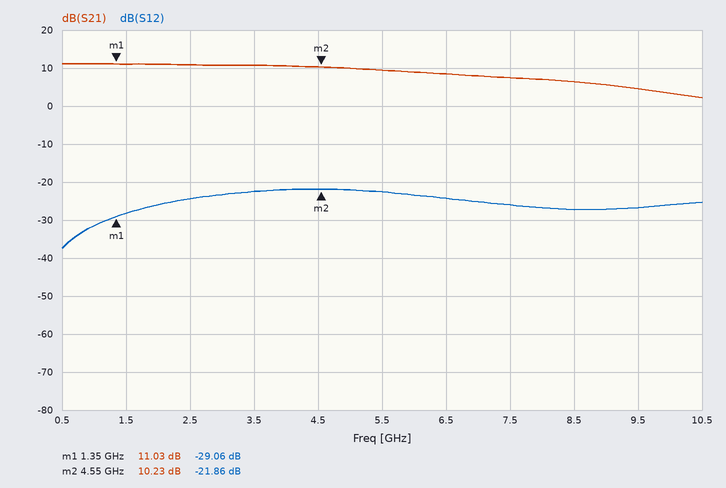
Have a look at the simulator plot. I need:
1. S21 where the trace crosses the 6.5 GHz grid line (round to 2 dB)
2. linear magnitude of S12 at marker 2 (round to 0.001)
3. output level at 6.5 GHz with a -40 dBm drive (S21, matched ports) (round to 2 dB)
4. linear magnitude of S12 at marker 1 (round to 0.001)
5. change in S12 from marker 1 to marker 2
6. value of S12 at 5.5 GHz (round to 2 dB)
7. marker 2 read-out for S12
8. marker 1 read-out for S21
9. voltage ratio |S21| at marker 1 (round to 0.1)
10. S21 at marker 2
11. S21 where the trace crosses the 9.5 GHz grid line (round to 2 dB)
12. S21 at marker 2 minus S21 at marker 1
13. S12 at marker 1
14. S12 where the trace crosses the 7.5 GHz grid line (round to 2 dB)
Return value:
8 dB
0.081
-32 dBm
0.035
7.20 dB
-22 dB
-21.86 dB
11.03 dB
3.6
10.23 dB
4 dB
-0.80 dB
-29.06 dB
-26 dB
